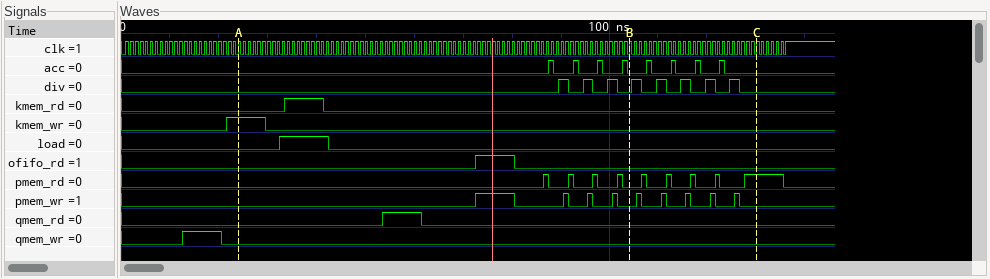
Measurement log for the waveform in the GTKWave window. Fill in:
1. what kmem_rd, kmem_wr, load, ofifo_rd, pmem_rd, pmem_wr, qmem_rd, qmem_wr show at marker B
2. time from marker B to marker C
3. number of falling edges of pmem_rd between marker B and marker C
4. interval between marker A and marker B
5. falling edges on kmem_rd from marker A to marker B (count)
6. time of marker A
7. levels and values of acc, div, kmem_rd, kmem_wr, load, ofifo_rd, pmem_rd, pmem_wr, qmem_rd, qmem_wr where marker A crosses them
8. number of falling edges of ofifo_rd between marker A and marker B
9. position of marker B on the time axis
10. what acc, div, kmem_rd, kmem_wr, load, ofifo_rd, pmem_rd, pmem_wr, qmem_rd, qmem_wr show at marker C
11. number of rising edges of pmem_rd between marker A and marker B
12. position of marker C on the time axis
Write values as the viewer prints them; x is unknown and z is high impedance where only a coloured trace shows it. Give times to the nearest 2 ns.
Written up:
kmem_rd=0, kmem_wr=0, load=0, ofifo_rd=0, pmem_rd=0, pmem_wr=0, qmem_rd=0, qmem_wr=0
26 ns
4
80 ns
1
24 ns
acc=0, div=0, kmem_rd=0, kmem_wr=1, load=0, ofifo_rd=0, pmem_rd=0, pmem_wr=0, qmem_rd=0, qmem_wr=0
1
104 ns
acc=0, div=0, kmem_rd=0, kmem_wr=0, load=0, ofifo_rd=0, pmem_rd=1, pmem_wr=0, qmem_rd=0, qmem_wr=0
4
130 ns
